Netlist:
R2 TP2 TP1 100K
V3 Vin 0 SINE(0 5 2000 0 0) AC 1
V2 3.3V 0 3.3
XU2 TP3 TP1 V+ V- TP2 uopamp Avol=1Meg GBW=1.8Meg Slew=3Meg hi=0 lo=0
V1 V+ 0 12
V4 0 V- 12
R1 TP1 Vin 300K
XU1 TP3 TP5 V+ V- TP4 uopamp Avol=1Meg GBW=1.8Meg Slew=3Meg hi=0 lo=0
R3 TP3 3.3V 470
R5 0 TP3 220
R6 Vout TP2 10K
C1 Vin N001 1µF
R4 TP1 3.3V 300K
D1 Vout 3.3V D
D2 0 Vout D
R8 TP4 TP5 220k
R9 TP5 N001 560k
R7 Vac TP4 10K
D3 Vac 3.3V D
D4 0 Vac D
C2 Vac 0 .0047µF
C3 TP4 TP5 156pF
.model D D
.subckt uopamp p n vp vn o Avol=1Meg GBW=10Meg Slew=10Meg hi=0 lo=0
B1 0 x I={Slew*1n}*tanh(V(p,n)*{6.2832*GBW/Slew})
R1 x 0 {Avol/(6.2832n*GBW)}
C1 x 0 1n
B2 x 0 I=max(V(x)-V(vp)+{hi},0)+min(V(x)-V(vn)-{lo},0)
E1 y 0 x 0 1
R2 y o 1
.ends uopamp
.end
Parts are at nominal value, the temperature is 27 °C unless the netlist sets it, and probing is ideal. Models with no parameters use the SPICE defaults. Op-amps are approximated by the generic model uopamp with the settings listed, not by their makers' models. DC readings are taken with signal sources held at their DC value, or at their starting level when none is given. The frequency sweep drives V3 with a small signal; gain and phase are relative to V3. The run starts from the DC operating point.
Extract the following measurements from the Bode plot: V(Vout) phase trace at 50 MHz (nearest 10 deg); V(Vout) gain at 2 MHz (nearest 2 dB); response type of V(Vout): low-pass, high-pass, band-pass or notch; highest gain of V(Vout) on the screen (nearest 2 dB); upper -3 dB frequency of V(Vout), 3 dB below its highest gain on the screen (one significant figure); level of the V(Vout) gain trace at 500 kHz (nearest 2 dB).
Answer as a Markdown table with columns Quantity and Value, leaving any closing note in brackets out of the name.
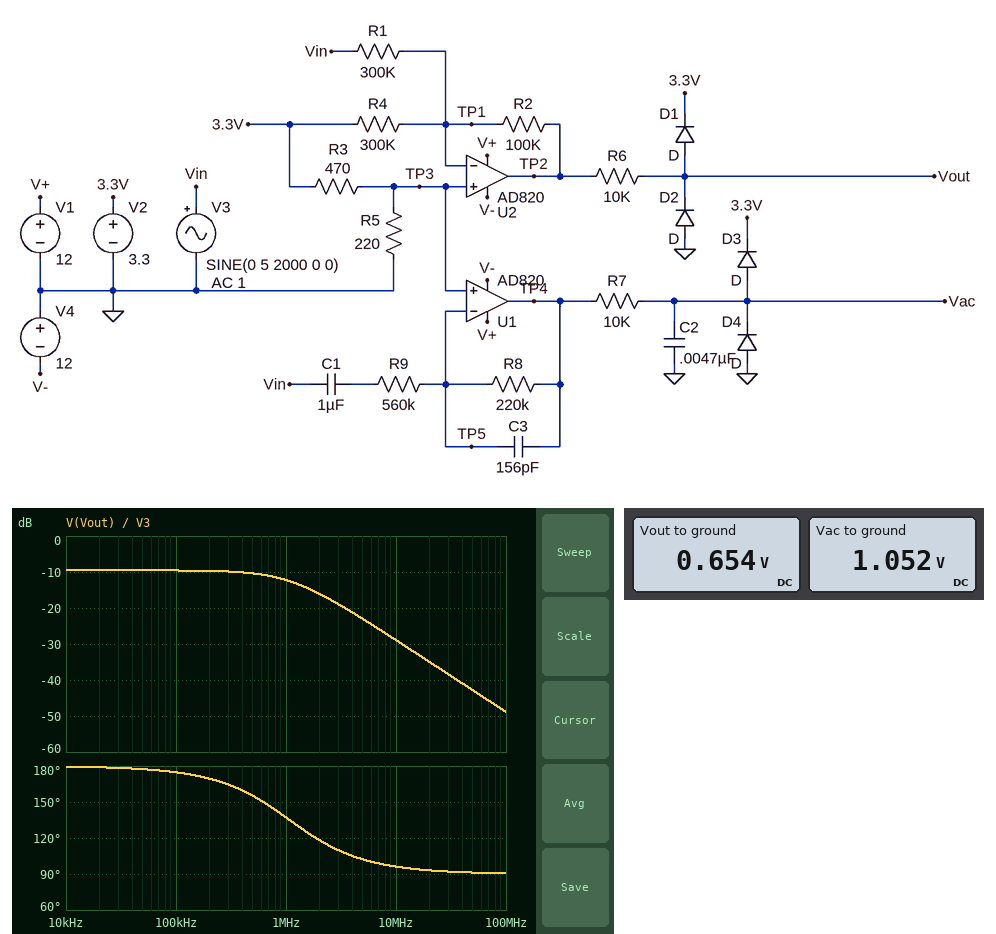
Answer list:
| Quantity | Value |
|---|---|
| V(Vout) phase trace at 50 MHz | 90 deg |
| V(Vout) gain at 2 MHz | -16 dB |
| response type of V(Vout): low-pass, high-pass, band-pass or notch | low-pass |
| highest gain of V(Vout) on the screen | -10 dB |
| upper -3 dB frequency of V(Vout), 3 dB below its highest gain on the screen | 1 MHz |
| level of the V(Vout) gain trace at 500 kHz | -10 dB |
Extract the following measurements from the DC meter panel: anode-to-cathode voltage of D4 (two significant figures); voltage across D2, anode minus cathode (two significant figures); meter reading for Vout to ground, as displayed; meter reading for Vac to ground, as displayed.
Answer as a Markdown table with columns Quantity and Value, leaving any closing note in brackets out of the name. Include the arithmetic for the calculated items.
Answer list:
| Quantity | Value |
|---|---|
| anode-to-cathode voltage of D4 | 0 V - 1.052 V = -1.1 V |
| voltage across D2, anode minus cathode | 0 V - 654 mV = -650 mV |
| meter reading for Vout to ground, as displayed | 0.654 V |
| meter reading for Vac to ground, as displayed | 1.052 V |
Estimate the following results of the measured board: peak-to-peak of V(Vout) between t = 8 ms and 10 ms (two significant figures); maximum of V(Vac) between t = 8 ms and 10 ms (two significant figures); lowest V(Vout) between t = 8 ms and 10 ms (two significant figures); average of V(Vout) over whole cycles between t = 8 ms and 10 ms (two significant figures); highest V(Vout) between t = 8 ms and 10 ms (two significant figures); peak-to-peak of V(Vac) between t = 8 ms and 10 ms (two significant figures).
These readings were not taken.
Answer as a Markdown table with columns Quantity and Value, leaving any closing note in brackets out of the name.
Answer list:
| Quantity | Value |
|---|---|
| peak-to-peak of V(Vout) between t = 8 ms and 10 ms | 2.9 V |
| maximum of V(Vac) between t = 8 ms and 10 ms | 2.6 V |
| lowest V(Vout) between t = 8 ms and 10 ms | -570 mV |
| average of V(Vout) over whole cycles between t = 8 ms and 10 ms | 730 mV |
| highest V(Vout) between t = 8 ms and 10 ms | 2.3 V |
| peak-to-peak of V(Vac) between t = 8 ms and 10 ms | 3.1 V |
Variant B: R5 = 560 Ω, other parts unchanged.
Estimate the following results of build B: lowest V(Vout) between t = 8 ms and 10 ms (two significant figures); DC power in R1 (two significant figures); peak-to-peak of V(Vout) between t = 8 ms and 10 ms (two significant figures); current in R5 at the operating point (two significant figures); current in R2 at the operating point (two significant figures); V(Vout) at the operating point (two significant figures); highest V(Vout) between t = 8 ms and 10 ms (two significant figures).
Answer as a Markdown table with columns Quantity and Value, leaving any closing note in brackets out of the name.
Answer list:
| Quantity | Value |
|---|---|
| lowest V(Vout) between t = 8 ms and 10 ms | 220 mV |
| DC power in R1 | 11 µW |
| peak-to-peak of V(Vout) between t = 8 ms and 10 ms | 3.3 V |
| current in R5 at the operating point | 3.2 mA |
| current in R2 at the operating point | 960 nA |
| V(Vout) at the operating point | 1.9 V |
| highest V(Vout) between t = 8 ms and 10 ms | 3.6 V |
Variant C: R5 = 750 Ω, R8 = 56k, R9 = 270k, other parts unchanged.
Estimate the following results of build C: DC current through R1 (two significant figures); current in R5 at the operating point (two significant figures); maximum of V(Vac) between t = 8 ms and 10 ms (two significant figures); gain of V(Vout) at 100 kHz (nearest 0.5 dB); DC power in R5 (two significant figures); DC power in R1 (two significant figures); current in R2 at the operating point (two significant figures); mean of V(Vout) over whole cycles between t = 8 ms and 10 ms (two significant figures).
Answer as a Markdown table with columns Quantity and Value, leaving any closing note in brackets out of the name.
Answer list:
| Quantity | Value |
|---|---|
| DC current through R1 | 6.8 µA |
| current in R5 at the operating point | 2.7 mA |
| maximum of V(Vac) between t = 8 ms and 10 ms | 2.9 V |
| gain of V(Vout) at 100 kHz | -9.5 dB |
| DC power in R5 | 5.5 mW |
| DC power in R1 | 14 µW |
| current in R2 at the operating point | 2.5 µA |
| mean of V(Vout) over whole cycles between t = 8 ms and 10 ms | 2.3 V |
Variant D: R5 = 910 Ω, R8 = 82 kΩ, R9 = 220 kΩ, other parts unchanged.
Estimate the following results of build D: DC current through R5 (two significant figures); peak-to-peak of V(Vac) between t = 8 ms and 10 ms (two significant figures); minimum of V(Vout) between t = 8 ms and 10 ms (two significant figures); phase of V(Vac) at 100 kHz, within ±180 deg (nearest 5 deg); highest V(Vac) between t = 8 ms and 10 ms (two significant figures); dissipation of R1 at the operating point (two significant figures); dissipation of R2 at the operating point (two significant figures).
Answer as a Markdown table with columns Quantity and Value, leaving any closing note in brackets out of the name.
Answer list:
| Quantity | Value |
|---|---|
| DC current through R5 | 2.4 mA |
| peak-to-peak of V(Vac) between t = 8 ms and 10 ms | 3.2 V |
| minimum of V(Vout) between t = 8 ms and 10 ms | 860 mV |
| phase of V(Vac) at 100 kHz, within ±180 deg | 5 deg |
| highest V(Vac) between t = 8 ms and 10 ms | 3.8 V |
| dissipation of R1 at the operating point | 16 µW |
| dissipation of R2 at the operating point | 1.2 µW |
